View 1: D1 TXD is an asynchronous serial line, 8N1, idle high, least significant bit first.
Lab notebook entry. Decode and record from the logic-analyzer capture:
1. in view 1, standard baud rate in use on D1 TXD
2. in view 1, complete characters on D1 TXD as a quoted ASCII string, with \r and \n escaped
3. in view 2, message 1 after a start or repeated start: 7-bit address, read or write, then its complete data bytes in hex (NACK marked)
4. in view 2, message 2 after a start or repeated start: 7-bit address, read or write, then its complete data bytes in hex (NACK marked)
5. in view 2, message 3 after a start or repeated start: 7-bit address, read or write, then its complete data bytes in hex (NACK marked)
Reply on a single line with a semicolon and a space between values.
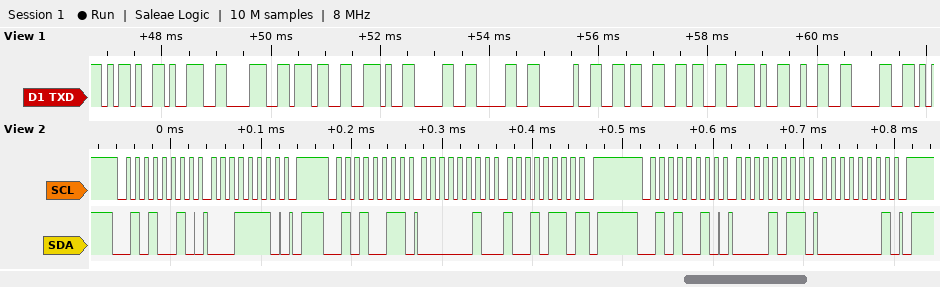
9600 baud; "-987.00 66.20"; 0x29 write: 1E; 0x29 read: 02 96 NACK; 0x29 write: 0B 01
